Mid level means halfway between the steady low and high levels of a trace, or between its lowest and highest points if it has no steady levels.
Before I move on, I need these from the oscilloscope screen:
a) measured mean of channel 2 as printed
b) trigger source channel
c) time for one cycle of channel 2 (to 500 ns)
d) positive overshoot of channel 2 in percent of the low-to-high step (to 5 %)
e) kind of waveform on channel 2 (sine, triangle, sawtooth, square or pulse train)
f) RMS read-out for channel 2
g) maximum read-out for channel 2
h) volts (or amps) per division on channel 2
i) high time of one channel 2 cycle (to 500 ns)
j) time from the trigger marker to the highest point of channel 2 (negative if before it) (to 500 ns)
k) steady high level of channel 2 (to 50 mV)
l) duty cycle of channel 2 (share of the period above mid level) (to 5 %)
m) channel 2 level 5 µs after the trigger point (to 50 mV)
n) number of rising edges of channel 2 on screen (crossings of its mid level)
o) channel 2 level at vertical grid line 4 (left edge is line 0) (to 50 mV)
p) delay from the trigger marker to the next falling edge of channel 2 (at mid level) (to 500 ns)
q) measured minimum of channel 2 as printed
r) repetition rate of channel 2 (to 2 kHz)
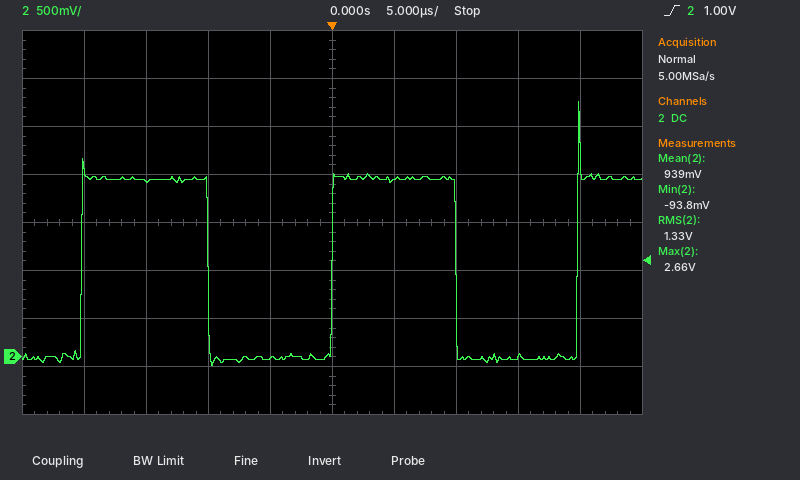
939 mV
channel 2
20.0 µs
45 %
square
1.33 V
2.66 V
500 mV
10.0 µs
+20.0 µs
1.85 V
50 %
1.85 V
3
0 mV
10.0 µs
-93.8 mV
50 kHz
